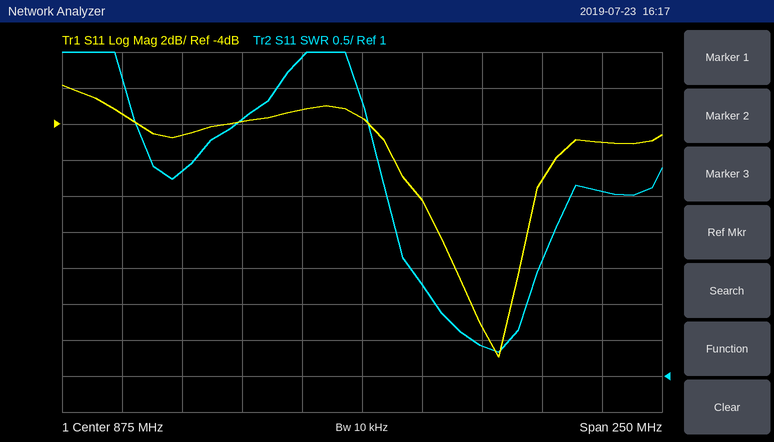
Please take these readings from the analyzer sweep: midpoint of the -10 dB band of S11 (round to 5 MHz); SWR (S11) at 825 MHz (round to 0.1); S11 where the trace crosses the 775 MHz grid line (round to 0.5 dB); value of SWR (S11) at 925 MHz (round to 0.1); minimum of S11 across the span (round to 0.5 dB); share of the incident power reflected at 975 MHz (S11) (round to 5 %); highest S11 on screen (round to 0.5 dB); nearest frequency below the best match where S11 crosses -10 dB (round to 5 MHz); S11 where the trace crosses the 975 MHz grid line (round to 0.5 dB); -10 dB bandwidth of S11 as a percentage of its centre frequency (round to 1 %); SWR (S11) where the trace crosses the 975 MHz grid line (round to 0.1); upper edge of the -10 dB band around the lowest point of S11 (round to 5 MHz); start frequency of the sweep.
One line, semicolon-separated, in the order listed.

925 MHz; 4.6; -3.5 dB; 1.4; -17.0 dB; 30 %; -2.0 dB; 905 MHz; -5.0 dB; 4 %; 3.6; 945 MHz; 750 MHz
